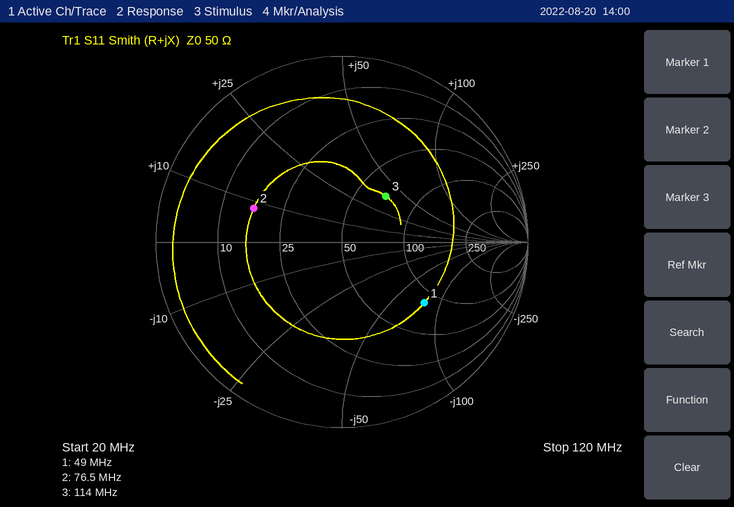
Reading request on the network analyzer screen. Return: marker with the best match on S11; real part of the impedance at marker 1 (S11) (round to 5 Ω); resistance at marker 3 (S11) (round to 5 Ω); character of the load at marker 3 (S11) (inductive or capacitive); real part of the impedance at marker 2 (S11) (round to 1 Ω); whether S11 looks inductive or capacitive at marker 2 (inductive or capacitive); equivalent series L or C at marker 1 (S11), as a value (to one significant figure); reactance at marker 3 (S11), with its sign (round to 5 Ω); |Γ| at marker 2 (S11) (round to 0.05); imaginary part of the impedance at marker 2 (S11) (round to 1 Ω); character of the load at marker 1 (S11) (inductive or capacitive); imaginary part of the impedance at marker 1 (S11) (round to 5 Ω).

marker 3
85 Ω
70 Ω
inductive
17 Ω
inductive
40 pF
+40 Ω
0.50
+8 Ω
capacitive
-80 Ω
